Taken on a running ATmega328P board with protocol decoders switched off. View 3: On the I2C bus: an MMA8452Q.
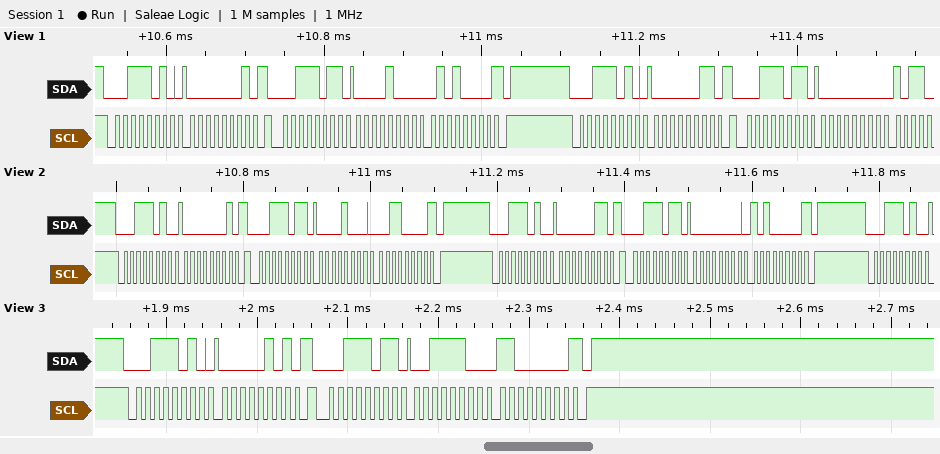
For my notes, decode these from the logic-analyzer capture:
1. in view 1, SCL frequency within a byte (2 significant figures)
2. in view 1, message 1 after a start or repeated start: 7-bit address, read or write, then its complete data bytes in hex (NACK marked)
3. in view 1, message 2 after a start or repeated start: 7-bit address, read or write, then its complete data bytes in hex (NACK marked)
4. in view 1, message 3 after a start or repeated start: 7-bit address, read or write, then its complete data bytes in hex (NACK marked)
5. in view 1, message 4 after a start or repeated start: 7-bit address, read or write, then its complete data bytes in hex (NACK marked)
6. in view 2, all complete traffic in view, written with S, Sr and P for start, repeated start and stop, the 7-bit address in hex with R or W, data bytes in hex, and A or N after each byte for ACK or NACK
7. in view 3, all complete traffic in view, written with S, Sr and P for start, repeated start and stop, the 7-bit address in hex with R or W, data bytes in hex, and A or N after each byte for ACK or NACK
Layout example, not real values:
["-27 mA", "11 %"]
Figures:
["100 kHz", "0x1D write: 01", "0x1D read: 08 50 NACK", "0x1D write: 03", "0x1D read: 00", "S 1DW A 01 A Sr 1DR A 08 A 30 N P S 1DW A 03 A Sr 1DR A 00 A A0 N P S 1DW A", "S 1DW A 05 A Sr 1DR A 3C A C0 N P"]
